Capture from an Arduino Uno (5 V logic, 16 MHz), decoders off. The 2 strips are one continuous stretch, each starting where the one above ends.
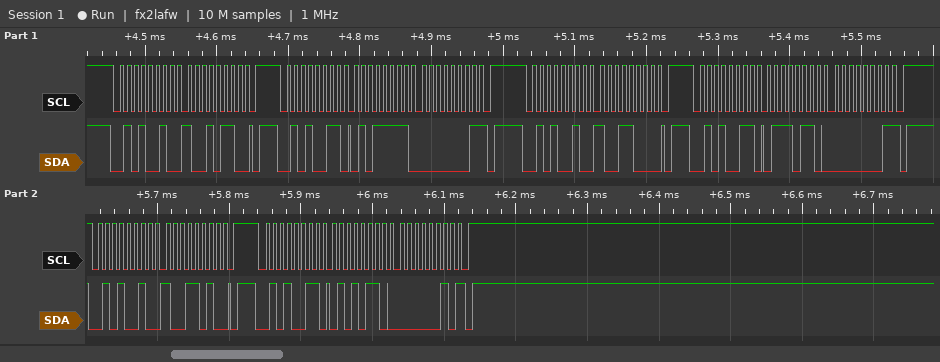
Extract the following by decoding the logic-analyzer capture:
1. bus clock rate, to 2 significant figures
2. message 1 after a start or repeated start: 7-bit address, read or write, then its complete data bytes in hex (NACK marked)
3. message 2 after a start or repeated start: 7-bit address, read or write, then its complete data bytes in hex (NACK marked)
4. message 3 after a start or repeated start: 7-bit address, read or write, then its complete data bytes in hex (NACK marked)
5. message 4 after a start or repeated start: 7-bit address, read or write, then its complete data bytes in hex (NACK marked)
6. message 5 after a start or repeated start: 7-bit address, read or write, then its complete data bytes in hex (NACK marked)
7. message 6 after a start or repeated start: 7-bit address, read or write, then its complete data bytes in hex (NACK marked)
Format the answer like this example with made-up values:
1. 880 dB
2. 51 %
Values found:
1. 100 kHz
2. 0x29 write: 96
3. 0x29 read: 5F 01 NACK
4. 0x29 write: 98
5. 0x29 read: 76 01 NACK
6. 0x29 write: 9A
7. 0x29 read: 56 02 NACK
